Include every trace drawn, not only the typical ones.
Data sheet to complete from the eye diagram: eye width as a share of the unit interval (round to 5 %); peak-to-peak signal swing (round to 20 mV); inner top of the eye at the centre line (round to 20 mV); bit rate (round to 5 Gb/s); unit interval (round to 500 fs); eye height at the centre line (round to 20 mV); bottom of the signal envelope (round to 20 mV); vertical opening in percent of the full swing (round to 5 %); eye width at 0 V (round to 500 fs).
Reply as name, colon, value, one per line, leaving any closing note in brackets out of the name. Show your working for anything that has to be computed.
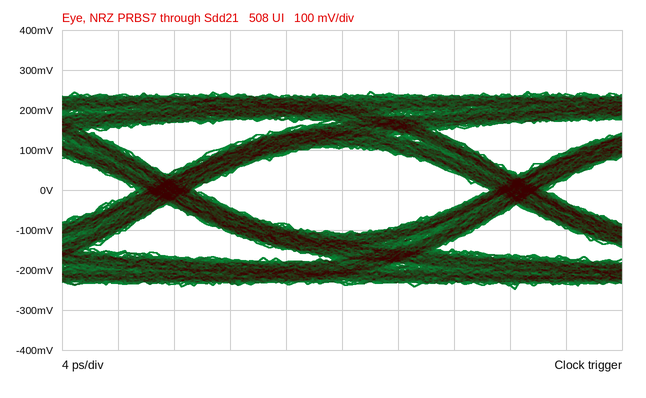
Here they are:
eye width as a share of the unit interval: 21.0 ps / 25.0 ps ≈ 84.0 %, so 85 % to the nearest 5 %
peak-to-peak signal swing: 500 mV
inner top of the eye at the centre line: 100 mV
bit rate: 40 Gb/s
unit interval: 25.0 ps
eye height at the centre line: 220 mV
bottom of the signal envelope: -240 mV
vertical opening in percent of the full swing: 220 mV / 500 mV ≈ 44.0 %, so 45 % to the nearest 5 %
eye width at 0 V: 21.0 ps
